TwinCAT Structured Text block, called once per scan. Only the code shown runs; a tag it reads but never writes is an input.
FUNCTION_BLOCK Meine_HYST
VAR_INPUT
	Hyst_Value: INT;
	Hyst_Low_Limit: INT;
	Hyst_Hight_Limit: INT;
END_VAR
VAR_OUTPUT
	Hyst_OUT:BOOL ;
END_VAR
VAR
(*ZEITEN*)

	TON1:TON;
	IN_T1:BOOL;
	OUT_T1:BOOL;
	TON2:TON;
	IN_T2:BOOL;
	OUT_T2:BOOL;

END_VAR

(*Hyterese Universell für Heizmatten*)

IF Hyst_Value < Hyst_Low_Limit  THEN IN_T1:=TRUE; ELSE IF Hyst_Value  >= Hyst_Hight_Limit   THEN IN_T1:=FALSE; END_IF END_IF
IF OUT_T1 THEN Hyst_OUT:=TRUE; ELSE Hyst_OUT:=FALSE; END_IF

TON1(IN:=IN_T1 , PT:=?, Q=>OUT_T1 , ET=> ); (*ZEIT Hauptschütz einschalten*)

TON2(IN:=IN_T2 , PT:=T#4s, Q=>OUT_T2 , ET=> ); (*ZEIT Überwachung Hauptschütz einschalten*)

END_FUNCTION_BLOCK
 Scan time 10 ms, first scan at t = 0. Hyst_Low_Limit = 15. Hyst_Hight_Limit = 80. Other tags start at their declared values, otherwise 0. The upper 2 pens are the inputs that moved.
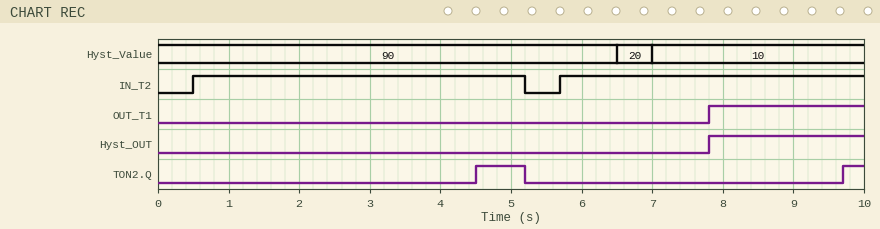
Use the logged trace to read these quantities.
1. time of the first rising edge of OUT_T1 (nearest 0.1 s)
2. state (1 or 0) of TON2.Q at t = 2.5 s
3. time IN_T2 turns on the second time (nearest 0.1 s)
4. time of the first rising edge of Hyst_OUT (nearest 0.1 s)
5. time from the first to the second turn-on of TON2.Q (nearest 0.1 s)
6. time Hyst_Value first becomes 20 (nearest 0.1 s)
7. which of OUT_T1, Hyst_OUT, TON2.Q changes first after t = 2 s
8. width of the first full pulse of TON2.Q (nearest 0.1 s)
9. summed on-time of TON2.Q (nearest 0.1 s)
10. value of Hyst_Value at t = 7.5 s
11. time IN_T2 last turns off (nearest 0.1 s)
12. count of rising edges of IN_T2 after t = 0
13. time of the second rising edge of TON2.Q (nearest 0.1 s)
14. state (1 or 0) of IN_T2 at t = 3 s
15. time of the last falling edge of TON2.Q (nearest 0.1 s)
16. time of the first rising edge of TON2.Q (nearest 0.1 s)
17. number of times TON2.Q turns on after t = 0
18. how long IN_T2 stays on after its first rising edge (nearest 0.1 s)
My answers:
7.8 s
0
5.7 s
7.8 s
5.2 s
6.5 s
TON2.Q
0.7 s
1.0 s
10
5.2 s
2
9.7 s
1
5.2 s
4.5 s
2
4.7 s
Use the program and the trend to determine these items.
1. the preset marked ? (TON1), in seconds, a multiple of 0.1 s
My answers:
0.8 s
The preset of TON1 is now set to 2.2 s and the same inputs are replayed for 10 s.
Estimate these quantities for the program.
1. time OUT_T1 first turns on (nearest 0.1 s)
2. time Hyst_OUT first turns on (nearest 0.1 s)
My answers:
9.2 s
9.2 s
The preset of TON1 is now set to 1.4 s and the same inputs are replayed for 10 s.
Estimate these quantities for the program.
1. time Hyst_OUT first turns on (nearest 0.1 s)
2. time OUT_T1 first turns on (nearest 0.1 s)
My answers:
8.4 s
8.4 s
